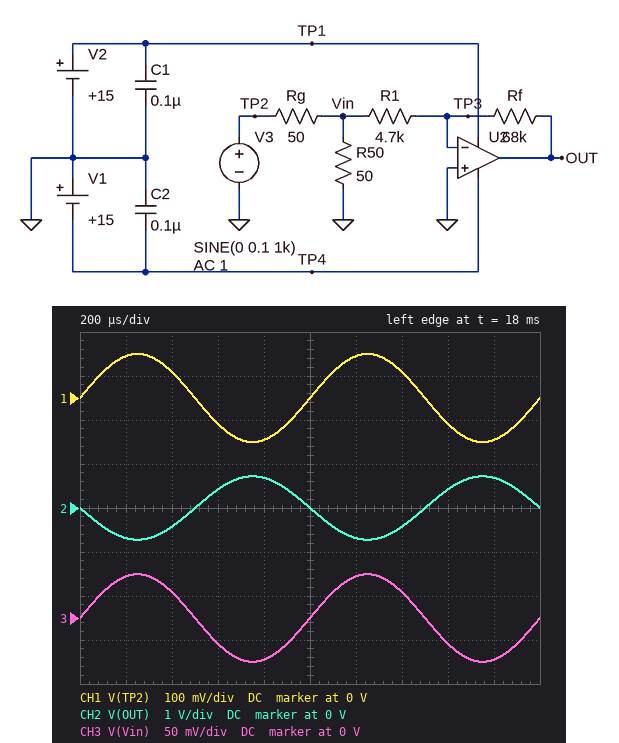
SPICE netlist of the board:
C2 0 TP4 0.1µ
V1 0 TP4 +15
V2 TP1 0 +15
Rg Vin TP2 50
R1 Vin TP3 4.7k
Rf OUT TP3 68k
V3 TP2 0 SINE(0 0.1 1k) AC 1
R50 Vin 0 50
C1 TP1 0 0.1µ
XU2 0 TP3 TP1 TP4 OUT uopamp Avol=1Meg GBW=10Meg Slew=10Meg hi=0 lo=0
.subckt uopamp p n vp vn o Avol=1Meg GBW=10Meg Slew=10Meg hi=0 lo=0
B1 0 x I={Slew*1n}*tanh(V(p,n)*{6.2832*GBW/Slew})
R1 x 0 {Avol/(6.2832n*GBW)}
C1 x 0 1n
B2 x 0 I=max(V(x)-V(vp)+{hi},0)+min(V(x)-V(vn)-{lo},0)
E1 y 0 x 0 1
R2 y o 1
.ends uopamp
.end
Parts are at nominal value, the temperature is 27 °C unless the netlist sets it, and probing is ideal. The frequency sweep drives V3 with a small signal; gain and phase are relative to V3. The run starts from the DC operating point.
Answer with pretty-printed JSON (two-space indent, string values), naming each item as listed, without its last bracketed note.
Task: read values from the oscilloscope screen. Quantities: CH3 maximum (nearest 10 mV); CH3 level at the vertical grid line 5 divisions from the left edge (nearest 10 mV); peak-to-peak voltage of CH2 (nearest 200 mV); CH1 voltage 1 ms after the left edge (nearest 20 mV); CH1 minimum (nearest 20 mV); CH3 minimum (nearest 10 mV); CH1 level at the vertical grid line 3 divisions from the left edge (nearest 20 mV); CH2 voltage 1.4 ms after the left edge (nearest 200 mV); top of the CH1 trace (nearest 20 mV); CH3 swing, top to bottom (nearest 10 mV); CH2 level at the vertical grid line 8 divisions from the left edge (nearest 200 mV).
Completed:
{
  "CH3 maximum": "50 mV",
  "CH3 level at the vertical grid line 5 divisions from the left edge": "0 V",
  "peak-to-peak voltage of CH2": "1.4 V",
  "CH1 voltage 1 ms after the left edge": "0 V",
  "CH1 minimum": "-100 mV",
  "CH3 minimum": "-50 mV",
  "CH1 level at the vertical grid line 3 divisions from the left edge": "-60 mV",
  "CH2 voltage 1.4 ms after the left edge": "-400 mV",
  "top of the CH1 trace": "100 mV",
  "CH3 swing, top to bottom": "100 mV",
  "CH2 level at the vertical grid line 8 divisions from the left edge": "400 mV"
}
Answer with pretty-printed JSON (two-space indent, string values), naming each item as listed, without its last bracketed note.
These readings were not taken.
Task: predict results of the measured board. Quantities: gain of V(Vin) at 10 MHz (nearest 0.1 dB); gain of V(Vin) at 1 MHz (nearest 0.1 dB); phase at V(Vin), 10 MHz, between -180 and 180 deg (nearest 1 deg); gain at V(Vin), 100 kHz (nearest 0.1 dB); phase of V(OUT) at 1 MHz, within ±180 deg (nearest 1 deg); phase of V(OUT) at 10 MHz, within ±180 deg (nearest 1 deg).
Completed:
{
  "gain of V(Vin) at 10 MHz": "-6.0 dB",
  "gain of V(Vin) at 1 MHz": "-6.0 dB",
  "phase at V(Vin), 10 MHz, between -180 and 180 deg": "0 deg",
  "gain at V(Vin), 100 kHz": "-6.1 dB",
  "phase of V(OUT) at 1 MHz, within ±180 deg": "123 deg",
  "phase of V(OUT) at 10 MHz, within ±180 deg": "94 deg"
}
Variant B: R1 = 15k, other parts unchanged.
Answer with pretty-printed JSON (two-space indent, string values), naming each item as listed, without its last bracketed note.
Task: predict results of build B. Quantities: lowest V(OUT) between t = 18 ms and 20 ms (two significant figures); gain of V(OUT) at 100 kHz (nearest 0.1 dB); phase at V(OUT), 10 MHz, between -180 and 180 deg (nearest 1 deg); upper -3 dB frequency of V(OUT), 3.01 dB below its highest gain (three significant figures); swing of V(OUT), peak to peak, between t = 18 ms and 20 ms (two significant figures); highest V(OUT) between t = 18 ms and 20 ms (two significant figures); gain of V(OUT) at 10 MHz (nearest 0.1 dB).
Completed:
{
  "lowest V(OUT) between t = 18 ms and 20 ms": "-230 mV",
  "gain of V(OUT) at 100 kHz": "7.1 dB",
  "phase at V(OUT), 10 MHz, between -180 and 180 deg": "100 deg",
  "upper -3 dB frequency of V(OUT), 3.01 dB below its highest gain": "1.81 MHz",
  "swing of V(OUT), peak to peak, between t = 18 ms and 20 ms": "450 mV",
  "highest V(OUT) between t = 18 ms and 20 ms": "230 mV",
  "gain of V(OUT) at 10 MHz": "-7.9 dB"
}
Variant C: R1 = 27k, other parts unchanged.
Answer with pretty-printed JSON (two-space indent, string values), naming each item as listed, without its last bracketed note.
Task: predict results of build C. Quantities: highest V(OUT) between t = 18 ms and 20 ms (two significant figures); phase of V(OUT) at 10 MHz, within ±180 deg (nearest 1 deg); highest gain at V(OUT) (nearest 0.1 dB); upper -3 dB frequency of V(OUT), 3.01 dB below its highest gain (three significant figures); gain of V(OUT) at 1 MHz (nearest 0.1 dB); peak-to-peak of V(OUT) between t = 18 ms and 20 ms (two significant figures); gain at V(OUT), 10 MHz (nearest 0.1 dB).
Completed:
{
  "highest V(OUT) between t = 18 ms and 20 ms": "130 mV",
  "phase of V(OUT) at 10 MHz, within ±180 deg": "106 deg",
  "highest gain at V(OUT)": "2.0 dB",
  "upper -3 dB frequency of V(OUT), 3.01 dB below its highest gain": "2.84 MHz",
  "gain of V(OUT) at 1 MHz": "1.5 dB",
  "peak-to-peak of V(OUT) between t = 18 ms and 20 ms": "250 mV",
  "gain at V(OUT), 10 MHz": "-9.3 dB"
}
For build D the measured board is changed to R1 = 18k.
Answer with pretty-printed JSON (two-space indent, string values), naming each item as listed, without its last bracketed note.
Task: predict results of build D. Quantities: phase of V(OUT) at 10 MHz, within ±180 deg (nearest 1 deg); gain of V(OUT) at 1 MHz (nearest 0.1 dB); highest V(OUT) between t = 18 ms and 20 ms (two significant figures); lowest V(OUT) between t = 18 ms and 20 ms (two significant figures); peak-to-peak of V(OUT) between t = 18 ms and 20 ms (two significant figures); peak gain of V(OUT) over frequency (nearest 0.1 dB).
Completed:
{
  "phase of V(OUT) at 10 MHz, within ±180 deg": "102 deg",
  "gain of V(OUT) at 1 MHz": "4.6 dB",
  "highest V(OUT) between t = 18 ms and 20 ms": "190 mV",
  "lowest V(OUT) between t = 18 ms and 20 ms": "-190 mV",
  "peak-to-peak of V(OUT) between t = 18 ms and 20 ms": "380 mV",
  "peak gain of V(OUT) over frequency": "5.5 dB"
}
